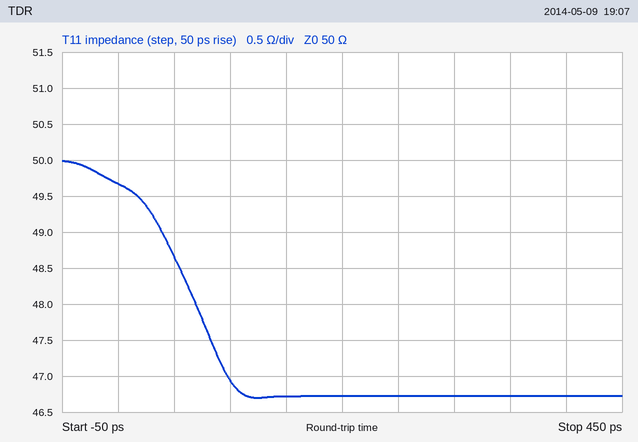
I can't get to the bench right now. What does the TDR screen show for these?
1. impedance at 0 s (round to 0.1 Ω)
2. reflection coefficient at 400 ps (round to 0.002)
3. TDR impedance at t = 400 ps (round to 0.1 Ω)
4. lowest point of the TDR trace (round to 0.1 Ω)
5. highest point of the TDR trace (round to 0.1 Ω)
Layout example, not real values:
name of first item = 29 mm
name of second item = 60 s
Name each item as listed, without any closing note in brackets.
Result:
impedance at 0 s = 49.7 Ω
reflection coefficient at 400 ps = -0.034
TDR impedance at t = 400 ps = 46.7 Ω
lowest point of the TDR trace = 46.7 Ω
highest point of the TDR trace = 50.0 Ω
